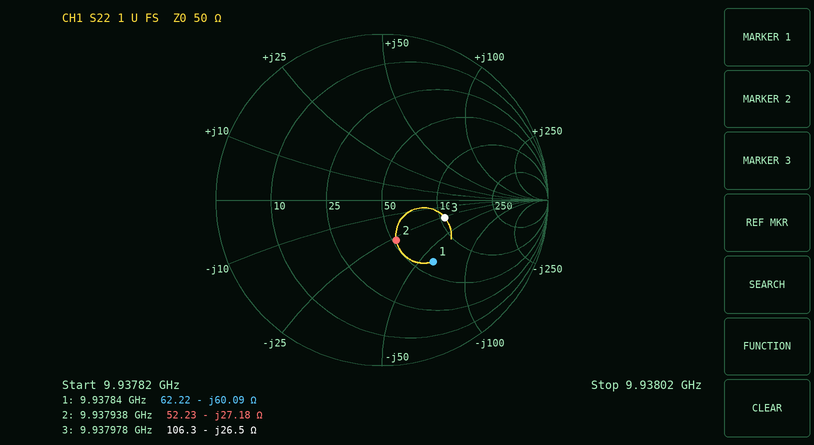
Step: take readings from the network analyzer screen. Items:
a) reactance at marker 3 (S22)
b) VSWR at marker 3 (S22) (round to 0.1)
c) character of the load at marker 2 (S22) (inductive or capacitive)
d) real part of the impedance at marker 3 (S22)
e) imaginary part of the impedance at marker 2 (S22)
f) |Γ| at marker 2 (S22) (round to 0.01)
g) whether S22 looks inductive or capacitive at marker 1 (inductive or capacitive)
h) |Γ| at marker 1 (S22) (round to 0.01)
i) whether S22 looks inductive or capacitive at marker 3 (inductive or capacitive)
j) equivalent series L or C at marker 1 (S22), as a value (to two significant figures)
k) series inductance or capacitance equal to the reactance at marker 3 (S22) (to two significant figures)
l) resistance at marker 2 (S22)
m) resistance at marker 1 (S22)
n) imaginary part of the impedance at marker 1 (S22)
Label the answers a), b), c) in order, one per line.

a) -26.5 Ω
b) 2.3
c) capacitive
d) 106.3 Ω
e) -27.18 Ω
f) 0.26
g) capacitive
h) 0.48
i) capacitive
j) 270 fF
k) 600 fF
l) 52.23 Ω
m) 62.22 Ω
n) -60.09 Ω
